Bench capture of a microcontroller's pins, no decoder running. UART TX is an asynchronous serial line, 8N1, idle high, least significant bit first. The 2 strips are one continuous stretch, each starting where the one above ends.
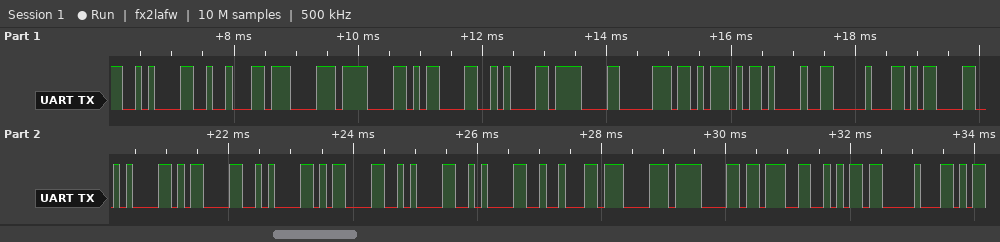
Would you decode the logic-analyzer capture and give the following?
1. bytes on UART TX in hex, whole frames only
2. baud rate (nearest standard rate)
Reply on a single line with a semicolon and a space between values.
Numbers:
0A 12 87 0F 0D 0A 0F 70 5D 21 10 0D 0A 0D 0A 0D 0A 0A 12 87 0F 3B 6A 10; 9600 baud
